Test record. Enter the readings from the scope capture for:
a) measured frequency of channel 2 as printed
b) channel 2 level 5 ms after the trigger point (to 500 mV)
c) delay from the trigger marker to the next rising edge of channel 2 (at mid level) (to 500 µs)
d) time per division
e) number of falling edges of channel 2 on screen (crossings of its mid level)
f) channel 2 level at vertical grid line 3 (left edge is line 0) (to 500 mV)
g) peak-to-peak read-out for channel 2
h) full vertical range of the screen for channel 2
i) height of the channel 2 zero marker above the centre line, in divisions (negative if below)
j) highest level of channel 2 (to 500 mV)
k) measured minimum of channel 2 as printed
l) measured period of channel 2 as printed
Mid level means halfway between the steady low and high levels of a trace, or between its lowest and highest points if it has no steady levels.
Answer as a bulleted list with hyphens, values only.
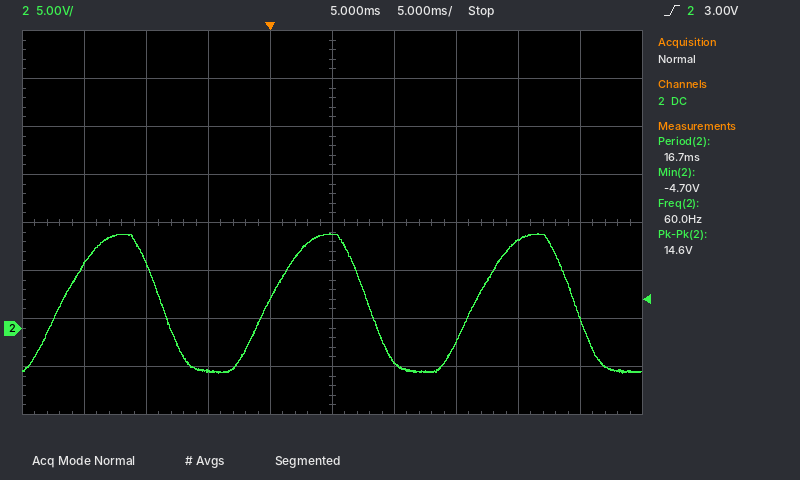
- 60.0 Hz
- 10.0 V
- 16.5 ms
- 5 ms
- 3
- -4.5 V
- 14.6 V
- 40 V
- -2.2 div
- 10.0 V
- -4.70 V
- 16.7 ms
